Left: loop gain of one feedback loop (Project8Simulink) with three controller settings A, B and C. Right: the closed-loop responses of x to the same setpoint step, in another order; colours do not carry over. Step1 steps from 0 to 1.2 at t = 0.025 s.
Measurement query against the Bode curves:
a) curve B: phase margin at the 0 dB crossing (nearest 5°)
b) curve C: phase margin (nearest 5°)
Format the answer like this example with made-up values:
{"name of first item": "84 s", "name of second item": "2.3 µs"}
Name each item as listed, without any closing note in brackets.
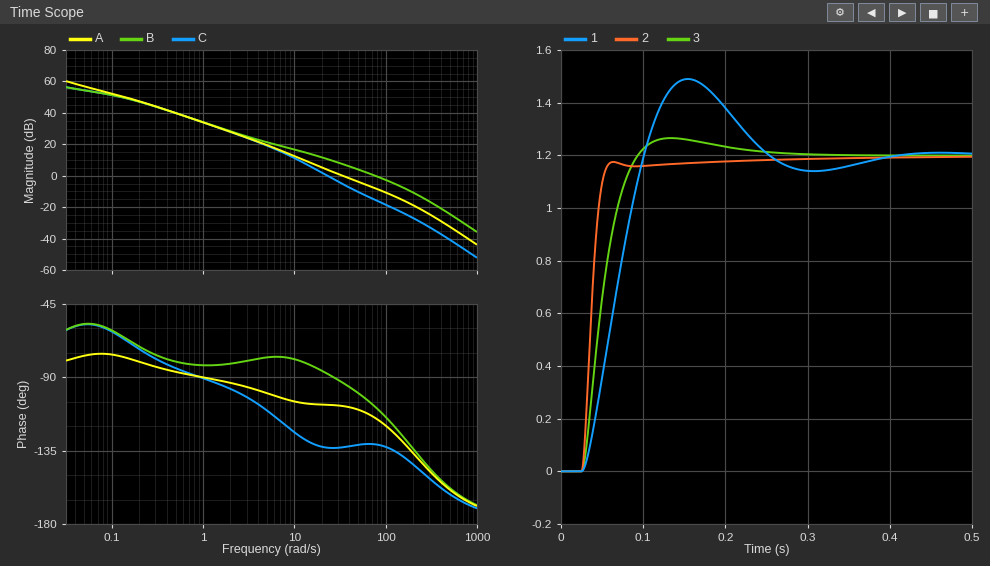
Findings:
{"curve B: phase margin at the 0 dB crossing": "70°", "curve C: phase margin": "45°"}
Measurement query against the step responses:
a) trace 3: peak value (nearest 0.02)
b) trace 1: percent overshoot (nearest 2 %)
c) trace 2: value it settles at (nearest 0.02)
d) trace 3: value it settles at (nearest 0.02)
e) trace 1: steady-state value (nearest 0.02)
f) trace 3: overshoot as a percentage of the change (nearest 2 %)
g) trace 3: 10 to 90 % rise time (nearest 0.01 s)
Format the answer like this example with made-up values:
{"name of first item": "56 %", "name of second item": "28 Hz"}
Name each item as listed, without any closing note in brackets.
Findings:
{"trace 3: peak value": "1.26", "trace 1: percent overshoot": "24 %", "trace 2: value it settles at": "1.20", "trace 3: value it settles at": "1.20", "trace 1: steady-state value": "1.20", "trace 3: overshoot as a percentage of the change": "6 %", "trace 3: 10 to 90 % rise time": "0.04 s"}
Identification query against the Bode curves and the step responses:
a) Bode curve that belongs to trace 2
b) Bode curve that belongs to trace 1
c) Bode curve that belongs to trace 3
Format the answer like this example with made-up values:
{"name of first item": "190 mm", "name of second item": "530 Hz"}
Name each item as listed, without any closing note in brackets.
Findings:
{"Bode curve that belongs to trace 2": "B", "Bode curve that belongs to trace 1": "C", "Bode curve that belongs to trace 3": "A"}
